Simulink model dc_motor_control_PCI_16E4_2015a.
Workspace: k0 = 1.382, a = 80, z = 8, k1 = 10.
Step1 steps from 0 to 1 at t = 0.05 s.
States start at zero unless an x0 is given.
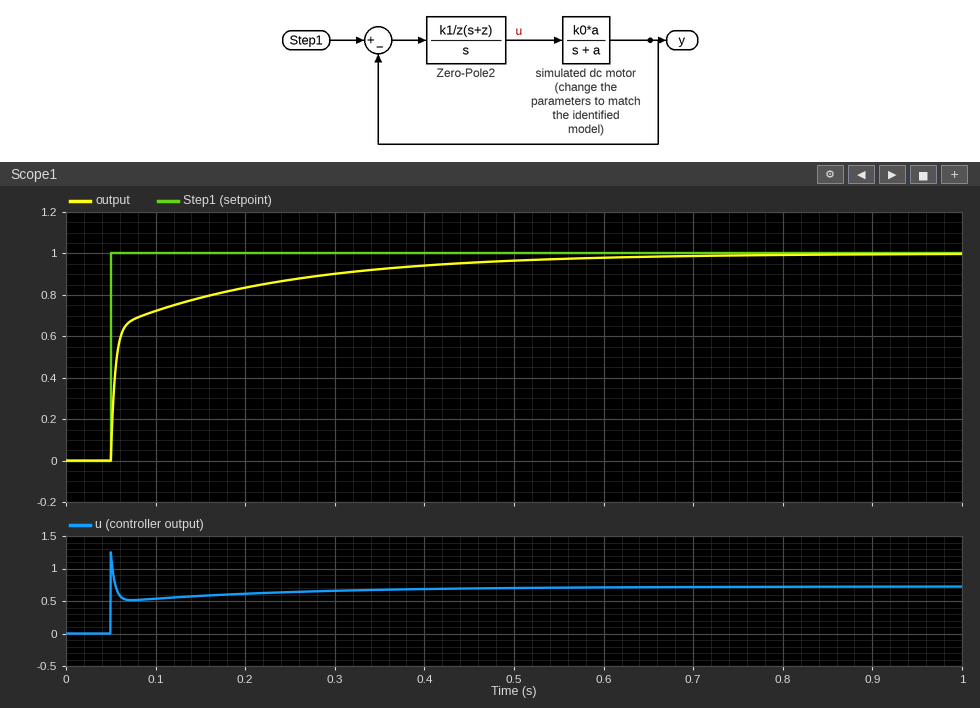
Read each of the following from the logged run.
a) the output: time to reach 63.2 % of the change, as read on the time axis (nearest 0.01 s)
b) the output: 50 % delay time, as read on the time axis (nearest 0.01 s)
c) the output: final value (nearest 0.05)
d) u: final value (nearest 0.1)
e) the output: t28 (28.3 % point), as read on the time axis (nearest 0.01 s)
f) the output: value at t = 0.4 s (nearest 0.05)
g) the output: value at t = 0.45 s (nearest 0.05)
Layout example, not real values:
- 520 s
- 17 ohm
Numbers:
- 0.06 s
- 0.06 s
- 1.00
- 0.7
- 0.05 s
- 0.95
- 0.95
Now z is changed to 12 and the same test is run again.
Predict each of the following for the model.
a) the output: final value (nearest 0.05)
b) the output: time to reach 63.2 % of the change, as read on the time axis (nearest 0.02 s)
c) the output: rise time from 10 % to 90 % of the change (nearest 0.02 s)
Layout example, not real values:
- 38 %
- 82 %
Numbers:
- 1.00
- 0.08 s
- 0.22 s
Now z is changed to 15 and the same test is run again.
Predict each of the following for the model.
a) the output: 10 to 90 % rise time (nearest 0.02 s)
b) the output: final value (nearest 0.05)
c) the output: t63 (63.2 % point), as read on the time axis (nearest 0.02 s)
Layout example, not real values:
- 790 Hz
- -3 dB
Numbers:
- 0.22 s
- 1.00
- 0.10 s
